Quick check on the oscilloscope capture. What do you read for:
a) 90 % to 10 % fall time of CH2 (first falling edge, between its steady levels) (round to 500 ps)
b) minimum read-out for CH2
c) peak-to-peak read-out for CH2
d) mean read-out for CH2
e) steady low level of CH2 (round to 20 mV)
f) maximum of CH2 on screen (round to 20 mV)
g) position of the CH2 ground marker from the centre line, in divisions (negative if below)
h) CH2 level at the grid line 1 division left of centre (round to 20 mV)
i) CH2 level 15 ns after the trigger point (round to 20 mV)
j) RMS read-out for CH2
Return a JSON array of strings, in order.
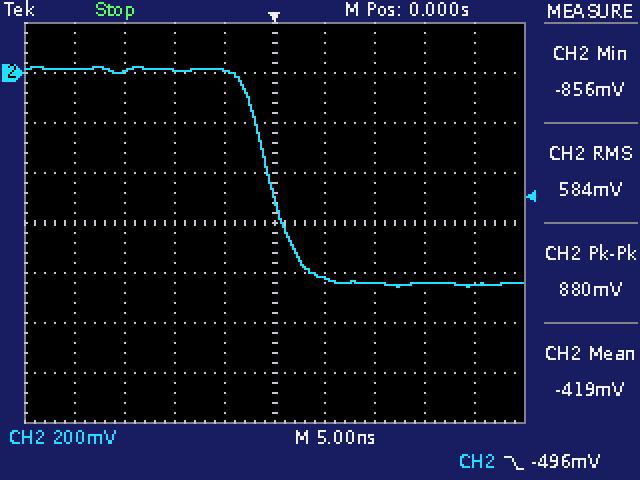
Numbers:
["5.5 ns", "-856 mV", "880 mV", "-419 mV", "-840 mV", "20 mV", "+3.0 div", "20 mV", "-840 mV", "584 mV"]
